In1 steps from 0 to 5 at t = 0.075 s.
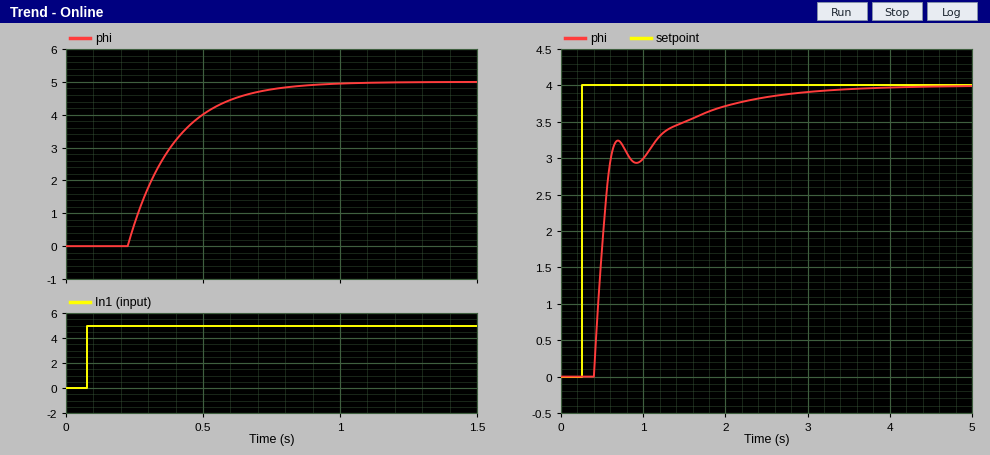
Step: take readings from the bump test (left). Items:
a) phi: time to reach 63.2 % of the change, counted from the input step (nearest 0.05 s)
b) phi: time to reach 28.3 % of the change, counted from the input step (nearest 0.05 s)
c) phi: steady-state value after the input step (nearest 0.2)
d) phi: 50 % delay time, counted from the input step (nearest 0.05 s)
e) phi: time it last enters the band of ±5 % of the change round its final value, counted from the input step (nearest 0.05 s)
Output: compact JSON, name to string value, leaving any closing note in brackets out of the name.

{"phi: time to reach 63.2 % of the change, counted from the input step": "0.30 s", "phi: time to reach 28.3 % of the change, counted from the input step": "0.20 s", "phi: steady-state value after the input step": "5.0", "phi: 50 % delay time, counted from the input step": "0.25 s", "phi: time it last enters the band of ±5 % of the change round its final value, counted from the input step": "0.65 s"}
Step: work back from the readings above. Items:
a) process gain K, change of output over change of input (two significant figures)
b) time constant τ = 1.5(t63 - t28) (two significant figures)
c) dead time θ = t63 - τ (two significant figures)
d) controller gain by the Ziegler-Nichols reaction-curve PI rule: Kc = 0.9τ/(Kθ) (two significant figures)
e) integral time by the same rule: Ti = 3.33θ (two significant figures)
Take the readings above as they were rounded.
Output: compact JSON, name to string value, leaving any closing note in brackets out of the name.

{"process gain K, change of output over change of input": "1.0", "time constant τ = 1.5(t63 - t28)": "0.15 s", "dead time θ = t63 - τ": "0.15 s", "controller gain by the Ziegler-Nichols reaction-curve PI rule: Kc = 0.9τ/(Kθ)": "0.90", "integral time by the same rule: Ti = 3.33θ": "0.50 s"}
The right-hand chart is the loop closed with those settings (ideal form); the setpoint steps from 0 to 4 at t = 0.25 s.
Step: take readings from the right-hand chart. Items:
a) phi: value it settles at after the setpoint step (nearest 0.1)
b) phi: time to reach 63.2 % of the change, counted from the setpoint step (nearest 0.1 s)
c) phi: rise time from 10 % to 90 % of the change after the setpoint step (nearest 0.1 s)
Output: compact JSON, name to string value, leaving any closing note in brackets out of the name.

{"phi: value it settles at after the setpoint step": "4.0", "phi: time to reach 63.2 % of the change, counted from the setpoint step": "0.3 s", "phi: rise time from 10 % to 90 % of the change after the setpoint step": "1.3 s"}
